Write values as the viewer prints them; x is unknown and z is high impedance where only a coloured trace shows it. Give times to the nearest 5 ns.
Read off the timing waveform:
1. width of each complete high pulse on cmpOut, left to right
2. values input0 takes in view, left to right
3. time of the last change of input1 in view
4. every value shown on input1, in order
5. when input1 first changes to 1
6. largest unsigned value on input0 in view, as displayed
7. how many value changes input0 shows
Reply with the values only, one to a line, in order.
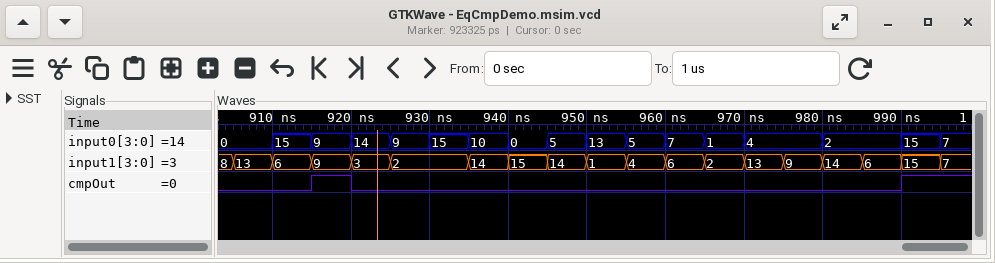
5 ns
0, 15, 9, 14, 9, 15, 10, 0, 5, 13, 5, 7, 1, 4, 2, 15, 7
995 ns
8, 13, 6, 9, 3, 2, 14, 15, 14, 1, 4, 6, 2, 13, 9, 14, 6, 15, 7
950 ns
15
16
